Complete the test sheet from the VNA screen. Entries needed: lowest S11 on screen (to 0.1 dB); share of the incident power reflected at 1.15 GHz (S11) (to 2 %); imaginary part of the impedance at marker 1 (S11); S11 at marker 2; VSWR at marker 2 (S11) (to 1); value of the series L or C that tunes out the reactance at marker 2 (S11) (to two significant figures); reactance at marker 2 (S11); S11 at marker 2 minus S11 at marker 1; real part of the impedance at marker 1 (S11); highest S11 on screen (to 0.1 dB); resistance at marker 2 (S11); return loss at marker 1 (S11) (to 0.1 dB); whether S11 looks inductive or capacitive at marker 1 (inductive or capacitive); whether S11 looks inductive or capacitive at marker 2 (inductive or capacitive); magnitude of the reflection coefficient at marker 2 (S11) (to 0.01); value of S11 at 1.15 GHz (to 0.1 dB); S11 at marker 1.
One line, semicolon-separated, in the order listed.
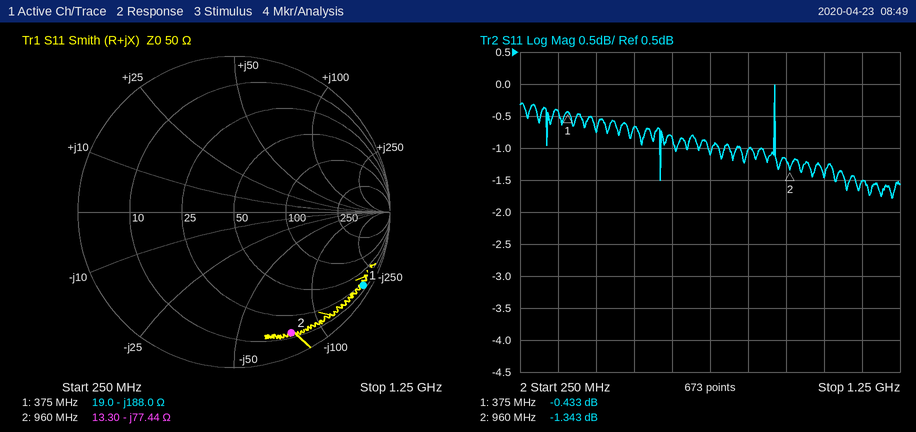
-1.8 dB; 70 %; -188.0 Ω; -1.343 dB; 13; 13 nH; -77.44 Ω; -0.910 dB; 19.0 Ω; 0.0 dB; 13.30 Ω; 0.4 dB; capacitive; capacitive; 0.86; -1.5 dB; -0.433 dB
